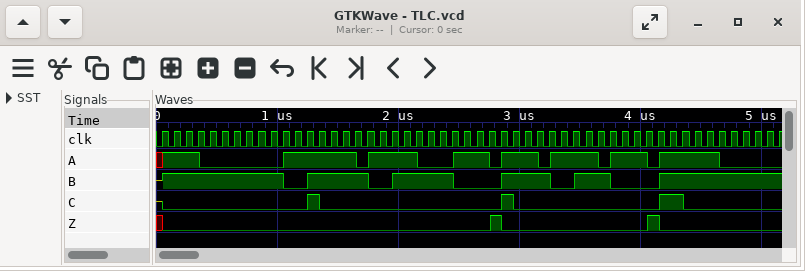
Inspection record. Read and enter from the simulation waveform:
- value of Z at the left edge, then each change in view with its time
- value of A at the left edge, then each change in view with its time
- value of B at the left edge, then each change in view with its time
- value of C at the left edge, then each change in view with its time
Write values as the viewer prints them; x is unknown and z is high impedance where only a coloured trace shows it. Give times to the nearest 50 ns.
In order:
x, 0 at 50 ns, 1 at 2750 ns, 0 at 2850 ns, 1 at 4050 ns, 0 at 4150 ns
x, 1 at 50 ns, 0 at 350 ns, 1 at 1050 ns, 0 at 1650 ns, 1 at 1750 ns, 0 at 2150 ns, 1 at 2450 ns, 0 at 2750 ns, 1 at 2850 ns, 0 at 3150 ns, 1 at 3250 ns, 0 at 3650 ns, 1 at 3750 ns, 0 at 4050 ns, 1 at 4150 ns, 0 at 4650 ns
z, 1 at 50 ns, 0 at 1050 ns, 1 at 1250 ns, 0 at 1750 ns, 1 at 1950 ns, 0 at 2450 ns, 1 at 2850 ns, 0 at 3250 ns, 1 at 3450 ns, 0 at 3750 ns, 1 at 4150 ns
z, 0 at 50 ns, 1 at 1250 ns, 0 at 1350 ns, 1 at 2850 ns, 0 at 2950 ns, 1 at 4150 ns, 0 at 4350 ns
